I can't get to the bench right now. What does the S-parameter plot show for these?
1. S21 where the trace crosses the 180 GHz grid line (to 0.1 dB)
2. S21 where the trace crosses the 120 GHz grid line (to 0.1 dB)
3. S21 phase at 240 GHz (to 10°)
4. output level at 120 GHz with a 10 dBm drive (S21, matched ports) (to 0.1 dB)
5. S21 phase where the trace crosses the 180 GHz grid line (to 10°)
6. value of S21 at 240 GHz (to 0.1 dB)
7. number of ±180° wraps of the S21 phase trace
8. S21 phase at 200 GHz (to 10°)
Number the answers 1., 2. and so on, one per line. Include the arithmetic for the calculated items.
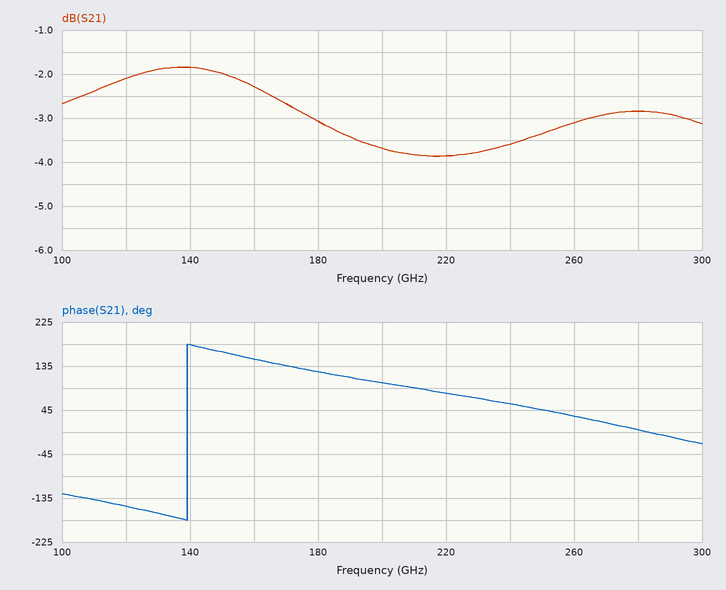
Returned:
1. -3.1 dB
2. -2.1 dB
3. 60°
4. 10 dBm + (-2.1 dB) = 7.9 dBm
5. 120°
6. -3.6 dB
7. 1
8. 100°
